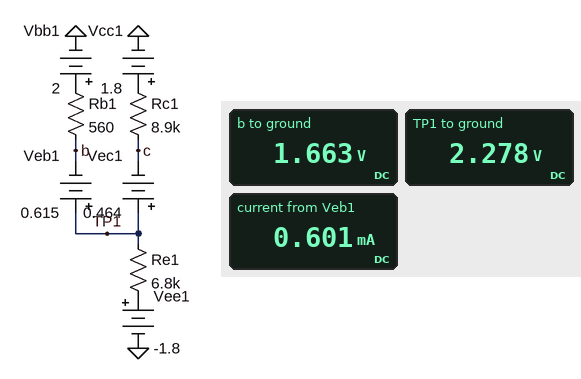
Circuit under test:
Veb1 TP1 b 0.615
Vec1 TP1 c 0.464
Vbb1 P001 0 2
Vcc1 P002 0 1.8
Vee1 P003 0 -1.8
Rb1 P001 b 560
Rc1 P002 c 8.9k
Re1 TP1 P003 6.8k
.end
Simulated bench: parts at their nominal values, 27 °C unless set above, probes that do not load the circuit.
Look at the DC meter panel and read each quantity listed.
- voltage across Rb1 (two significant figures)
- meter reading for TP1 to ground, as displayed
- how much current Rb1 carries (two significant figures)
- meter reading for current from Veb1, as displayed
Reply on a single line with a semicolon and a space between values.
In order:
340 mV; 2.278 V; 600 µA; 0.601 mA
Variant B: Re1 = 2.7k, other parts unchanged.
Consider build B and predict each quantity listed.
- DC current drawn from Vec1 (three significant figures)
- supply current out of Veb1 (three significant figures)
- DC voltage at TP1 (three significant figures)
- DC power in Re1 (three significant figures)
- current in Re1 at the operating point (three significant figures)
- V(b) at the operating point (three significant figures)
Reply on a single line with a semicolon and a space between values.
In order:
43.5 µA; 1.32 mA; 1.88 V; 5.01 mW; 1.36 mA; 1.26 V
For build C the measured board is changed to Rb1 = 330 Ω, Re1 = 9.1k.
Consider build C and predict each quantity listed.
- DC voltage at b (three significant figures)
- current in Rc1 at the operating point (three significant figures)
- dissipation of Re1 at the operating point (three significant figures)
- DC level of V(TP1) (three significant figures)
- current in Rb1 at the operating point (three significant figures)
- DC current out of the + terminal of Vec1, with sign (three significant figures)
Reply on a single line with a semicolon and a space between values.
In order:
1.84 V; 21.3 µA; 1.99 mW; 2.45 V; 489 µA; -21.3 µA
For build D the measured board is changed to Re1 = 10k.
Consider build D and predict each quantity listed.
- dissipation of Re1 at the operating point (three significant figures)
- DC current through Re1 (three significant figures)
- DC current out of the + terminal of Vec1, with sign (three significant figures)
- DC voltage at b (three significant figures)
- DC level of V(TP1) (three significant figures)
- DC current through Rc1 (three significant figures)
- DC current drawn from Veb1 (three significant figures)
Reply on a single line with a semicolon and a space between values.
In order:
1.74 mW; 417 µA; -12.4 µA; 1.76 V; 2.37 V; 12.4 µA; 430 µA
